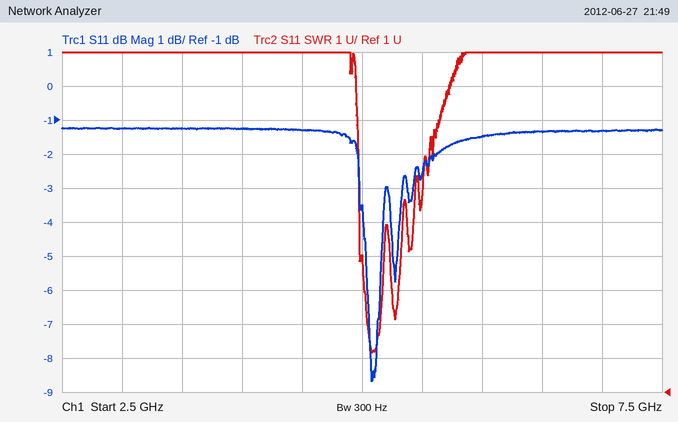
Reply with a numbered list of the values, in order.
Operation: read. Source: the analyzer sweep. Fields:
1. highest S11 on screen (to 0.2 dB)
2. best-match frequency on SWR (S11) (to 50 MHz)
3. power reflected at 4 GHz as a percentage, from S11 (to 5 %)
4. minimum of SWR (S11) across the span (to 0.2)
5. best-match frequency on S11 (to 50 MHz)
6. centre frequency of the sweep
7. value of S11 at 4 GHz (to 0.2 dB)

1. -1.2 dB
2. 5.10 GHz
3. 75 %
4. 2.2
5. 5.10 GHz
6. 5 GHz
7. -1.2 dB
